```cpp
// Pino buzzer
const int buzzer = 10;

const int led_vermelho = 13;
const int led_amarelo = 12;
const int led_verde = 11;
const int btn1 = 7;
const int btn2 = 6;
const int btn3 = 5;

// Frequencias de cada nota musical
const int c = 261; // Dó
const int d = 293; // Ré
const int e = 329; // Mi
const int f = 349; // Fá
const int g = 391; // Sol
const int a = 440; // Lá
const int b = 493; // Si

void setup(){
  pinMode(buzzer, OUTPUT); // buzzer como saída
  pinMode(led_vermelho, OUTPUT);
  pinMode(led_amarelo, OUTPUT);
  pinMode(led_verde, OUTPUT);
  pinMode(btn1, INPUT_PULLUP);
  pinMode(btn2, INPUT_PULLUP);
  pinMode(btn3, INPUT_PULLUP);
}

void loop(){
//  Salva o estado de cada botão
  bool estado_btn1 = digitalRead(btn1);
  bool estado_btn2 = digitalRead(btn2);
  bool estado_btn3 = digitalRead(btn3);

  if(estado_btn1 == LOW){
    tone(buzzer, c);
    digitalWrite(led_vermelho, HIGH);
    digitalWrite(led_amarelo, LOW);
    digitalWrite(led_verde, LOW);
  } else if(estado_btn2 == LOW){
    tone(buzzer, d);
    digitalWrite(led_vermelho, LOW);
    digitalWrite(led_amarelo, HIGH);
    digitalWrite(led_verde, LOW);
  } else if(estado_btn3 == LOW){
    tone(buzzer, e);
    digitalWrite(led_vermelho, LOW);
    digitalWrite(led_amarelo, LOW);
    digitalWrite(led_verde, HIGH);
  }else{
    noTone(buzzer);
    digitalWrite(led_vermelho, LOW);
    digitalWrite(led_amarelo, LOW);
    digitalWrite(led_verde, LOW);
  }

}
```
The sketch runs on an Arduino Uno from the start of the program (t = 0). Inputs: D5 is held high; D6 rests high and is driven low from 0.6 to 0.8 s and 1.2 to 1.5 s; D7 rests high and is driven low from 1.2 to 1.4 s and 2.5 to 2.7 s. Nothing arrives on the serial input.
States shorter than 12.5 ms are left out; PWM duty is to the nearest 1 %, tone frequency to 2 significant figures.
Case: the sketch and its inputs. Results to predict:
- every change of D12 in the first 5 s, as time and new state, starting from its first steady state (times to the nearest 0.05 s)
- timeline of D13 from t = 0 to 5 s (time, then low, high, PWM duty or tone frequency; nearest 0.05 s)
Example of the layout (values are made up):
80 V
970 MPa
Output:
0 s low; 0.6 s high; 0.8 s low; 1.4 s high; 1.5 s low
0 s low; 1.2 s high; 1.4 s low; 2.5 s high; 2.7 s low
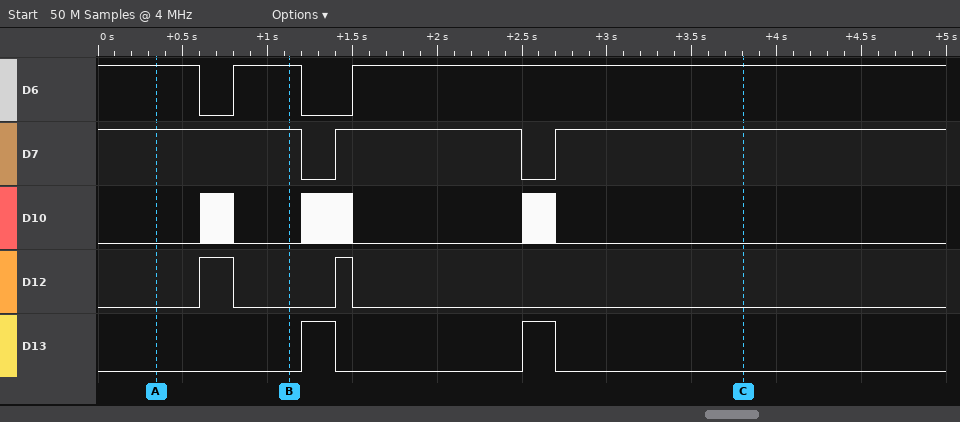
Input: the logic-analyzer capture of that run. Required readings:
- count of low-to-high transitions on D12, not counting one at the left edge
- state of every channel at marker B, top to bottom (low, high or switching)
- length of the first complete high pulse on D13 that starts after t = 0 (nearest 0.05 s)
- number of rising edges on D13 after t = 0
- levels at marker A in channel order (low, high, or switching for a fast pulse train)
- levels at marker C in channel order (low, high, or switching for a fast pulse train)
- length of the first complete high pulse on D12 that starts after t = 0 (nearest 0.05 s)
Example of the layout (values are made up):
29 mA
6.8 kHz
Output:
2
D6 high, D7 high, D10 low, D12 low, D13 low
0.20 s
2
D6 high, D7 high, D10 low, D12 low, D13 low
D6 high, D7 high, D10 low, D12 low, D13 low
0.20 s
